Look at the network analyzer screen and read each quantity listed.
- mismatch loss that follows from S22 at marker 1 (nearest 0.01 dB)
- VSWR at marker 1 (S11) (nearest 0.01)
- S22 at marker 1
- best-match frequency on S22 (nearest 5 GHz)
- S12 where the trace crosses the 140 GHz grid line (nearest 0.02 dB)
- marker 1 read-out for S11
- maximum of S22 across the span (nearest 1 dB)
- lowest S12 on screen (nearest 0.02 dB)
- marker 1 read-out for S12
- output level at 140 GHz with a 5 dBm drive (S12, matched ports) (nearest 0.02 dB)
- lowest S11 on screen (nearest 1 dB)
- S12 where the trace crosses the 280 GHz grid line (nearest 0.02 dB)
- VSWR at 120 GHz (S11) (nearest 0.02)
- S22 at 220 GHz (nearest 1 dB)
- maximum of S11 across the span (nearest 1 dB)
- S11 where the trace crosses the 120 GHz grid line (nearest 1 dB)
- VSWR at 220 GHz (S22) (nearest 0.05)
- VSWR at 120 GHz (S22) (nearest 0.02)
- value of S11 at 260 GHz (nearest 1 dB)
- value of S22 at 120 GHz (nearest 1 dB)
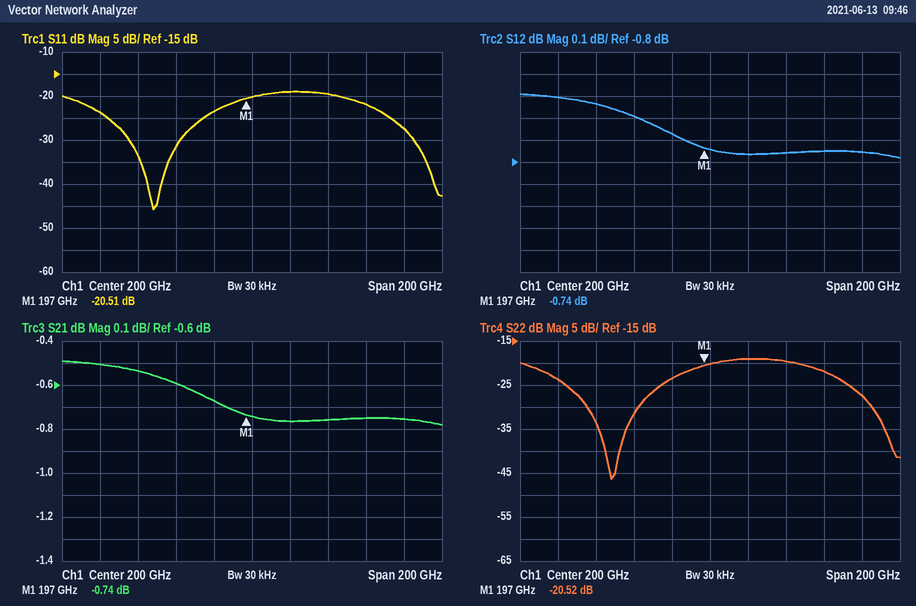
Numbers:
0.04 dB
1.21
-20.52 dB
150 GHz
-0.54 dB
-20.51 dB
-19 dB
-0.78 dB
-0.74 dB
4.46 dBm
-46 dB
-0.76 dB
1.14
-19 dB
-19 dB
-24 dB
1.25
1.14
-22 dB
-24 dB
